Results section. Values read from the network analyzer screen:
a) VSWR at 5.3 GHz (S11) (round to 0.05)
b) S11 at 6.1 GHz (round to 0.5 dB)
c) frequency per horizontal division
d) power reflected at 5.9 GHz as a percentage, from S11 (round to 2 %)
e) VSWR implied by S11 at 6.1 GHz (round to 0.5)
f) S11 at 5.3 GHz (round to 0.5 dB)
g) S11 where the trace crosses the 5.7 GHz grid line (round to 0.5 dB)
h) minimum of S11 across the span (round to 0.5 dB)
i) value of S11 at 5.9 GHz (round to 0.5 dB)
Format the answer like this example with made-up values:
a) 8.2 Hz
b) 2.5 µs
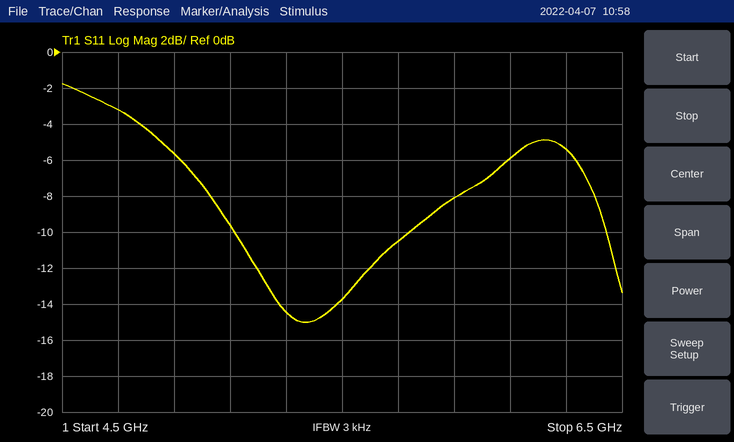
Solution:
a) 1.45
b) -6.0 dB
c) 200 MHz
d) 16 %
e) 3.0
f) -14.5 dB
g) -10.5 dB
h) -15.0 dB
i) -8.0 dB
